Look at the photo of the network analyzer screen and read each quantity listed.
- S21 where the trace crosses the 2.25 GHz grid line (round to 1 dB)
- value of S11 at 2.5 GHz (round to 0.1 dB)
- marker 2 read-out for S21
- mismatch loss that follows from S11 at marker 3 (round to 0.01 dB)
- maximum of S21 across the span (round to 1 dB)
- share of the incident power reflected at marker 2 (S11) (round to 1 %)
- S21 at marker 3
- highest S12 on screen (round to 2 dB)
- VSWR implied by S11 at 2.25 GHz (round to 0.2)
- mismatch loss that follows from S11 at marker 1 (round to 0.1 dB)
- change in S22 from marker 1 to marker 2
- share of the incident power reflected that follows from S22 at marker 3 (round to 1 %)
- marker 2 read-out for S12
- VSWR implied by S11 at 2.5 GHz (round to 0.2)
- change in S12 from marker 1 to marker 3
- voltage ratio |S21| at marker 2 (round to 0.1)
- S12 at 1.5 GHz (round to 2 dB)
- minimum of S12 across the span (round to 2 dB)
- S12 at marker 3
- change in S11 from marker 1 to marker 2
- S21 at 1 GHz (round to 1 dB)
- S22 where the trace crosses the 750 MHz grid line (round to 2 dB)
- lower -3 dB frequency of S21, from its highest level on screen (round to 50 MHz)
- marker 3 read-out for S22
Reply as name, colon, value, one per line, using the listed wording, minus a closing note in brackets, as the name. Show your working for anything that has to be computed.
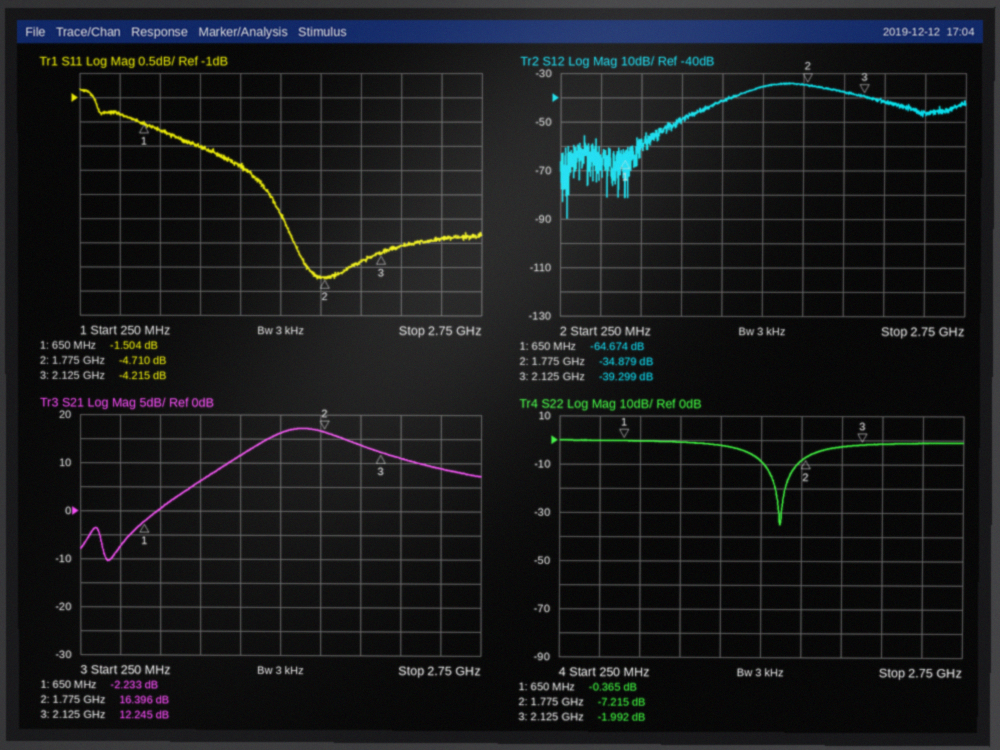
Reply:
S21 where the trace crosses the 2.25 GHz grid line: 11 dB
value of S11 at 2.5 GHz: -3.9 dB
marker 2 read-out for S21: 16.396 dB
mismatch loss that follows from S11 at marker 3: −10 log10(1 − 10^(-4.215/10)) ≈ 2.07 dB
maximum of S21 across the span: 17 dB
share of the incident power reflected at marker 2 (S11): 10^(-4.71/10) ≈ 34 %
S21 at marker 3: 12.245 dB
highest S12 on screen: -34 dB
VSWR implied by S11 at 2.25 GHz: |Γ| = 10^(-4.1/20) = 0.6237; VSWR = (1 + 0.6237)/(1 − 0.6237) ≈ 4.32, so 4.4 to the nearest 0.2
mismatch loss that follows from S11 at marker 1: −10 log10(1 − 10^(-1.504/10)) ≈ 5.3 dB
change in S22 from marker 1 to marker 2: -7.215 − (-0.365) = -6.850 dB
share of the incident power reflected that follows from S22 at marker 3: 10^(-1.992/10) ≈ 63 %
marker 2 read-out for S12: -34.879 dB
VSWR implied by S11 at 2.5 GHz: |Γ| = 10^(-3.9/20) = 0.6383; VSWR = (1 + 0.6383)/(1 − 0.6383) ≈ 4.53, so 4.6 to the nearest 0.2
change in S12 from marker 1 to marker 3: -39.299 − (-64.674) = 25.375 dB
voltage ratio |S21| at marker 2: 10^(16.396/20) ≈ 6.6
S12 at 1.5 GHz: -36 dB
minimum of S12 across the span: -90 dB
S12 at marker 3: -39.299 dB
change in S11 from marker 1 to marker 2: -4.71 − (-1.504) = -3.206 dB
S21 at 1 GHz: 6 dB
S22 where the trace crosses the 750 MHz grid line: 0 dB
lower -3 dB frequency of S21, from its highest level on screen: 1.40 GHz
marker 3 read-out for S22: -1.992 dB
